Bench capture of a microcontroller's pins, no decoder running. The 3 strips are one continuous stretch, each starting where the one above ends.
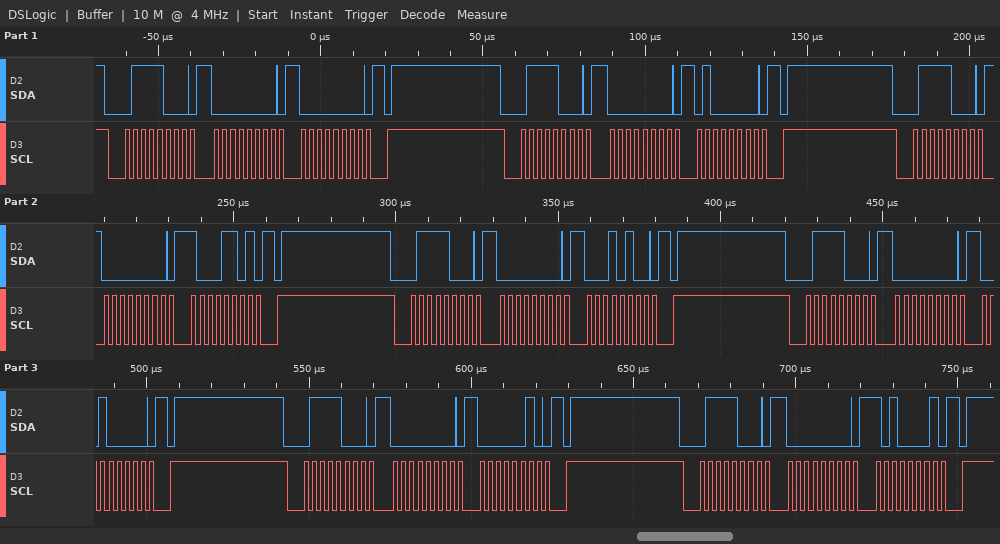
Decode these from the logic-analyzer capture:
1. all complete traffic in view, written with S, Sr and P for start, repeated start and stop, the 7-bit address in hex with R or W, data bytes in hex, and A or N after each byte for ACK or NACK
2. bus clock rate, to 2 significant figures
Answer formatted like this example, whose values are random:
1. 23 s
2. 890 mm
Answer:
1. S 3CW A 00 A 00 A P S 3CW A 00 A 40 A P S 3CW A 00 A 8D A P S 3CW A 00 A 14 A P S 3CW A 00 A 20 A P S 3CW A 00 A 02 A P S 3CW A 00 A A1 A P
2. 400 kHz
